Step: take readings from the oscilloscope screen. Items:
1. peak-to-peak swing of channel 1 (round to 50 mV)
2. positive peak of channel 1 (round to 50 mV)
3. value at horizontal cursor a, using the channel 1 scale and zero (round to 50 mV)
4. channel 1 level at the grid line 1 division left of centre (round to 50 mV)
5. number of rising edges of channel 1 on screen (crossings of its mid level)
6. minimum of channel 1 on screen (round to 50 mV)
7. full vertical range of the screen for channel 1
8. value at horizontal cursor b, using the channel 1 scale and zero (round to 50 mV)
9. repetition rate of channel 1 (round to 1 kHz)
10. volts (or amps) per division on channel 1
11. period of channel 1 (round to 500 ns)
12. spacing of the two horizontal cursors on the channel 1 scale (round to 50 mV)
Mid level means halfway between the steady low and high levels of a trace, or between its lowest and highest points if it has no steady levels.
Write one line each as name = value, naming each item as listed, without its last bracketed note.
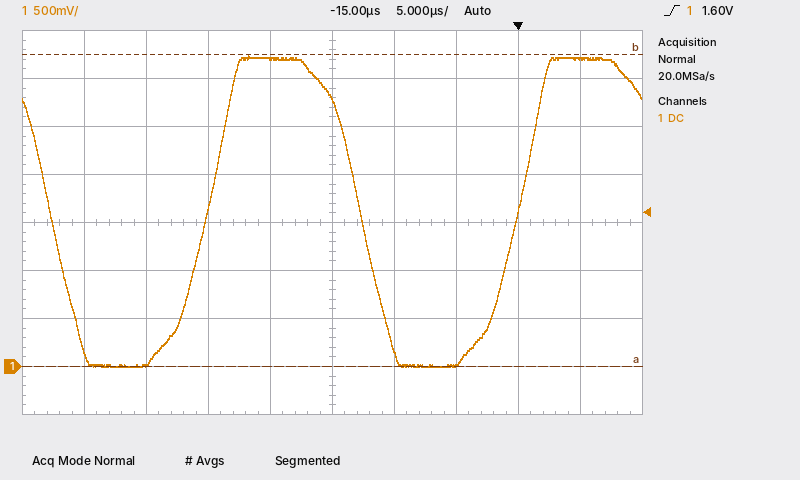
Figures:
peak-to-peak swing of channel 1 = 3.25 V
positive peak of channel 1 = 3.25 V
value at horizontal cursor a, using the channel 1 scale and zero = 0 mV
channel 1 level at the grid line 1 division left of centre = 3.20 V
number of rising edges of channel 1 on screen = 2
minimum of channel 1 on screen = 0 mV
full vertical range of the screen for channel 1 = 4 V
value at horizontal cursor b, using the channel 1 scale and zero = 3.25 V
repetition rate of channel 1 = 40 kHz
volts (or amps) per division on channel 1 = 500 mV
period of channel 1 = 25.0 µs
spacing of the two horizontal cursors on the channel 1 scale = 3.25 V
